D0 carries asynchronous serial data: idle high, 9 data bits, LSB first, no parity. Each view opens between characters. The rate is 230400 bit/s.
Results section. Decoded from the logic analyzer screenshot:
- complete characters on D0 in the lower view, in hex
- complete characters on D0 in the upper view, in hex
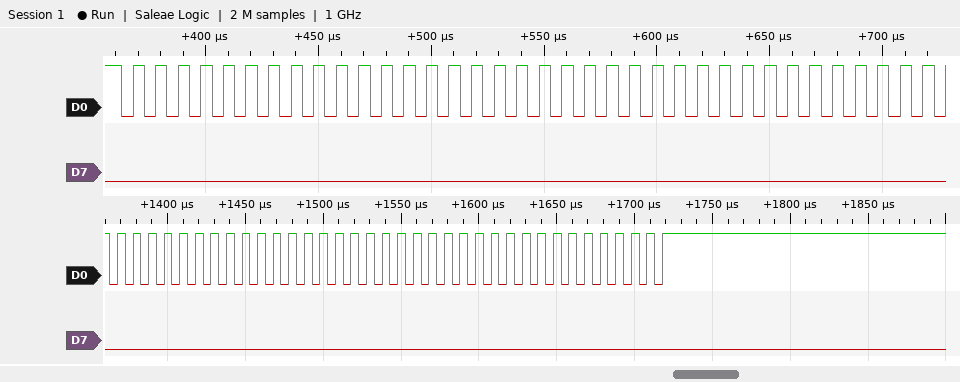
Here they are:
AD, AD, AD, AD, AD, AD, AD, 1FF
AD, AD, AD, AD, AD, AD, AD
